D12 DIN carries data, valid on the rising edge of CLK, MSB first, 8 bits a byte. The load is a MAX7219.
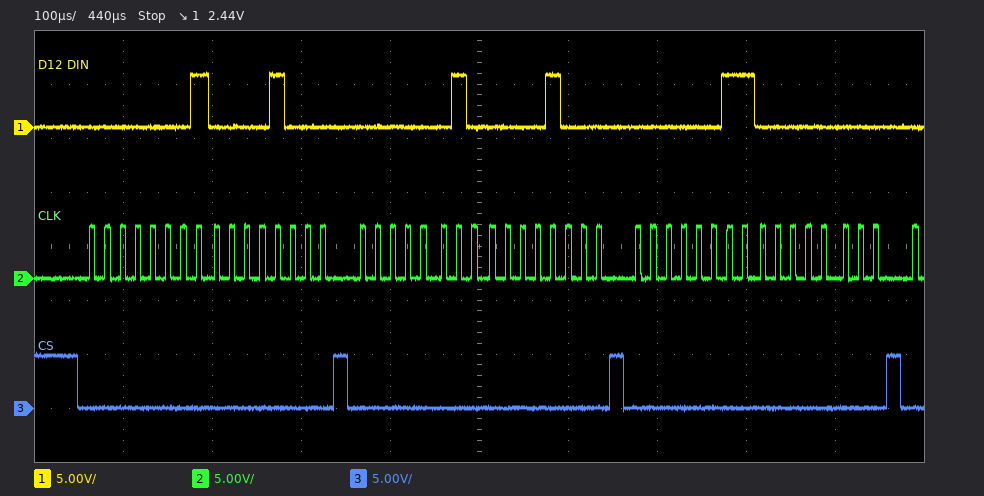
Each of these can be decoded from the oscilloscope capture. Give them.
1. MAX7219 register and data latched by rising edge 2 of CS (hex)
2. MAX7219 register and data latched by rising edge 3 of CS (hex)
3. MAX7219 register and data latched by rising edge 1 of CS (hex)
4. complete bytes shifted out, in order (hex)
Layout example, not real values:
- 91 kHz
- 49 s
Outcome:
- register 0x2, data 0x08
- register 0x3, data 0x00
- register 0x1, data 0x08
- 01 08 02 08 03 00
